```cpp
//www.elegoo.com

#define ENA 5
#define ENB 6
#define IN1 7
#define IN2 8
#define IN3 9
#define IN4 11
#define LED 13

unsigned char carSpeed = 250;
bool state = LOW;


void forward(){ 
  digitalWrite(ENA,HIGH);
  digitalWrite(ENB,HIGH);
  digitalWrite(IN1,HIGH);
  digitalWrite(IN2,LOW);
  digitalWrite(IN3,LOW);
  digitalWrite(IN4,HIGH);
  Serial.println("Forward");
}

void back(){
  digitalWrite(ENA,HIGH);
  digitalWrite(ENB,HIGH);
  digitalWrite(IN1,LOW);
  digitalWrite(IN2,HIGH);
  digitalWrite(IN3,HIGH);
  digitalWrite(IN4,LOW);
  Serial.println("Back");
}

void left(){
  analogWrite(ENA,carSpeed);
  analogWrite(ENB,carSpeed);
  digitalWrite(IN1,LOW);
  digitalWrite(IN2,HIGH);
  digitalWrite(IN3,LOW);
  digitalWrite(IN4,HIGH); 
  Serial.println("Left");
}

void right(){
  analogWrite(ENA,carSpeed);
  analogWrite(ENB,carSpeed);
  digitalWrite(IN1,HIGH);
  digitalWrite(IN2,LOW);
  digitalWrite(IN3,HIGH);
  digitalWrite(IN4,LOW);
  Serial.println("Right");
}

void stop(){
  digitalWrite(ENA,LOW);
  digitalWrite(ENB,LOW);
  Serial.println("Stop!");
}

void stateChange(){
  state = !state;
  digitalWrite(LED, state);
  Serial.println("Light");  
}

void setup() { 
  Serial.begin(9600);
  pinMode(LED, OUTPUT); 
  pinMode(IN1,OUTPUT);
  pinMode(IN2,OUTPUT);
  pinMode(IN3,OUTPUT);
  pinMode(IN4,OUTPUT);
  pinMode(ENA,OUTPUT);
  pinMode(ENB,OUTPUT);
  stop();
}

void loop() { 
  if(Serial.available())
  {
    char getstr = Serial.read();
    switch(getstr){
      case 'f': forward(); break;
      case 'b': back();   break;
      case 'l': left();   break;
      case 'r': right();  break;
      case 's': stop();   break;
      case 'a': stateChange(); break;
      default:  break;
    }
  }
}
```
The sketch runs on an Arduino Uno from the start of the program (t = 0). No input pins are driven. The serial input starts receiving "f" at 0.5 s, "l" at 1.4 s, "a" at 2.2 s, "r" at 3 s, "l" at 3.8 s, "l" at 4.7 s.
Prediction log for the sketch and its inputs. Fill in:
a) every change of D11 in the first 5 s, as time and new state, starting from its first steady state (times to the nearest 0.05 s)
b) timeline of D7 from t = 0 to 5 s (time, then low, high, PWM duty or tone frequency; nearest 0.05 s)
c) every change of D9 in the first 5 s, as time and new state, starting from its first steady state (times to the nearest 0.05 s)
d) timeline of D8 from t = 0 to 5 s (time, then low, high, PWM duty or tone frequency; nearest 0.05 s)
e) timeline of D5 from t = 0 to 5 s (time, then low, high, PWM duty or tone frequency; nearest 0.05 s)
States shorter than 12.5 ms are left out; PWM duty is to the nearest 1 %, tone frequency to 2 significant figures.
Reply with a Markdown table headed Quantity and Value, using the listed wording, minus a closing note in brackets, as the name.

| Quantity | Value |
|---|---|
| every change of D11 in the first 5 s, as time and new state, starting from its first steady state | 0 s low; 0.5 s high; 3 s low; 3.8 s high |
| timeline of D7 from t = 0 to 5 s | 0 s low; 0.5 s high; 1.4 s low; 3 s high; 3.8 s low |
| every change of D9 in the first 5 s, as time and new state, starting from its first steady state | 0 s low; 3 s high; 3.8 s low |
| timeline of D8 from t = 0 to 5 s | 0 s low; 1.4 s high; 3 s low; 3.8 s high |
| timeline of D5 from t = 0 to 5 s | 0 s low; 0.5 s high; 1.4 s PWM 98 % |
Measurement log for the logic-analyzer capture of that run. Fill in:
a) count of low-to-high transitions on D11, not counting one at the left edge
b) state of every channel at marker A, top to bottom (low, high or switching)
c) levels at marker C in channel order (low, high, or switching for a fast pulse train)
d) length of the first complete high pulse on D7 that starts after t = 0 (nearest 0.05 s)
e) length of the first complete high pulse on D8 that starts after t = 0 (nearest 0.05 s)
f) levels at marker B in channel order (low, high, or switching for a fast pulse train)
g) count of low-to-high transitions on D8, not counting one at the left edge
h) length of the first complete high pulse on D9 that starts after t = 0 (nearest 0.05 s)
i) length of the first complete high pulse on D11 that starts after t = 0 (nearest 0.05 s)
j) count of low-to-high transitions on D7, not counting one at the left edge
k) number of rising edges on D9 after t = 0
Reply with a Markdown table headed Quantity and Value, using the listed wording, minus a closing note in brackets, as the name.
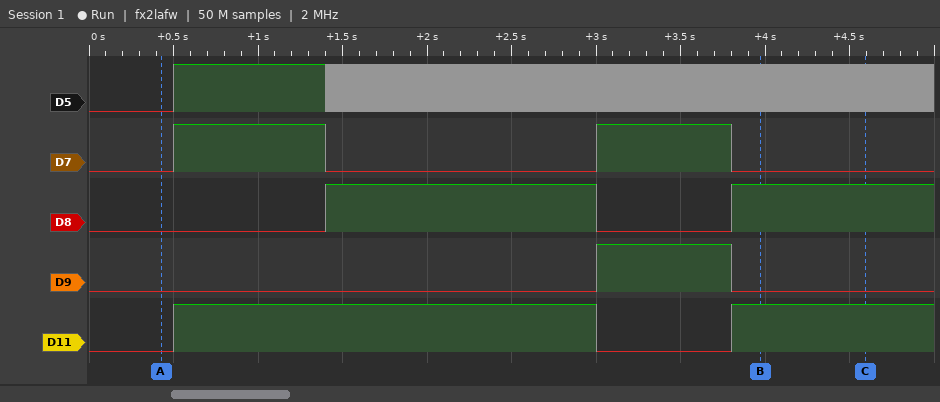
| Quantity | Value |
|---|---|
| count of low-to-high transitions on D11, not counting one at the left edge | 2 |
| state of every channel at marker A, top to bottom | D5 low, D7 low, D8 low, D9 low, D11 low |
| levels at marker C in channel order | D5 switching, D7 low, D8 high, D9 low, D11 high |
| length of the first complete high pulse on D7 that starts after t = 0 | 0.90 s |
| length of the first complete high pulse on D8 that starts after t = 0 | 1.60 s |
| levels at marker B in channel order | D5 switching, D7 low, D8 high, D9 low, D11 high |
| count of low-to-high transitions on D8, not counting one at the left edge | 2 |
| length of the first complete high pulse on D9 that starts after t = 0 | 0.80 s |
| length of the first complete high pulse on D11 that starts after t = 0 | 2.50 s |
| count of low-to-high transitions on D7, not counting one at the left edge | 2 |
| number of rising edges on D9 after t = 0 | 1 |
